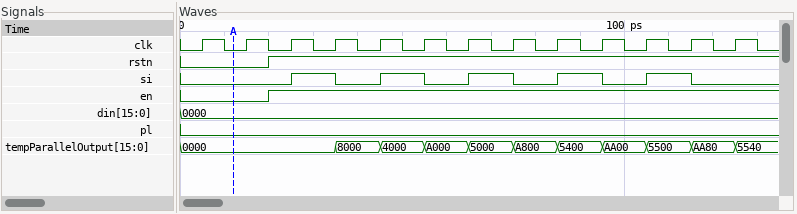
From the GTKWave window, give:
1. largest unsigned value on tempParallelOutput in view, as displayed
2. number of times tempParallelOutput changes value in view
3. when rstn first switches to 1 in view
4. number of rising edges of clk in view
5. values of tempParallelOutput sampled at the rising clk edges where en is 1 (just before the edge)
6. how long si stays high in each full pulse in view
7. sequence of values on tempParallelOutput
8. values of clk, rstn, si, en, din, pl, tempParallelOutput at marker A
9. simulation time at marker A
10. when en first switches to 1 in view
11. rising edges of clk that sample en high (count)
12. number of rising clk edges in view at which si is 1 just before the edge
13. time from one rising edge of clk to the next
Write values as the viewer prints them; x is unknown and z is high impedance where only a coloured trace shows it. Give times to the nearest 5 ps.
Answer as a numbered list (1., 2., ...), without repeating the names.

1. AA80
2. 10
3. 20 ps
4. 13
5. 0000, 0000, 8000, 4000, A000, 5000, A800, 5400, AA00, 5500, AA80
6. 10 ps, 10 ps, 10 ps, 10 ps, 10 ps
7. 0000, 8000, 4000, A000, 5000, A800, 5400, AA00, 5500, AA80, 5540
8. clk=0, rstn=0, si=0, en=0, din=0000, pl=0, tempParallelOutput=0000
9. 10 ps
10. 20 ps
11. 11
12. 5
13. 10 ps
